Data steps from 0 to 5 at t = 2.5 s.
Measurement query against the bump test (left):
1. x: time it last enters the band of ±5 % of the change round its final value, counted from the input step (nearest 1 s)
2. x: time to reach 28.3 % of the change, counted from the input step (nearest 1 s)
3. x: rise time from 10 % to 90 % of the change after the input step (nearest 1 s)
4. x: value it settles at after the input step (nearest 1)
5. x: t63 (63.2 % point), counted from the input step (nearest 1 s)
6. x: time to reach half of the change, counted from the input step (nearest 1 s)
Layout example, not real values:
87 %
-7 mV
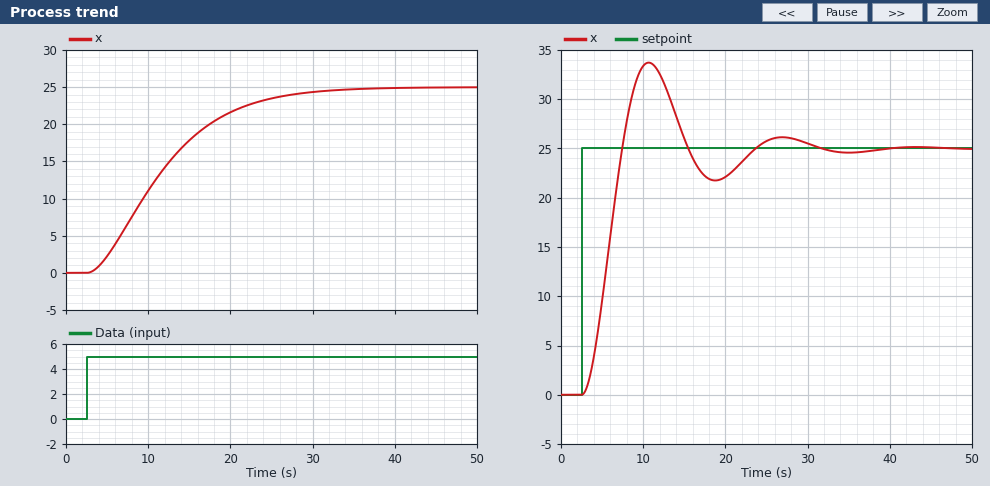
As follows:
24 s
5 s
17 s
25
11 s
8 s
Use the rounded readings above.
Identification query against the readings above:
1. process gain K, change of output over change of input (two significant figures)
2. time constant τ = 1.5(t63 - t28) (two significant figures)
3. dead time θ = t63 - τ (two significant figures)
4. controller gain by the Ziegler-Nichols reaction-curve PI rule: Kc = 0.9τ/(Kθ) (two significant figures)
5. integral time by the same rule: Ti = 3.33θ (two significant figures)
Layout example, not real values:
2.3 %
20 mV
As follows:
5.0
9.0 s
2.0 s
0.81
6.7 s
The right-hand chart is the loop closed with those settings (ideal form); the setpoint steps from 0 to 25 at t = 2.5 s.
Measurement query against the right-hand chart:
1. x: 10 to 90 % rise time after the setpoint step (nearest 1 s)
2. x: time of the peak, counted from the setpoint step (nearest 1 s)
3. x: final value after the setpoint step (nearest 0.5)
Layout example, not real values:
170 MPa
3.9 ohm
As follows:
3 s
8 s
25.0
